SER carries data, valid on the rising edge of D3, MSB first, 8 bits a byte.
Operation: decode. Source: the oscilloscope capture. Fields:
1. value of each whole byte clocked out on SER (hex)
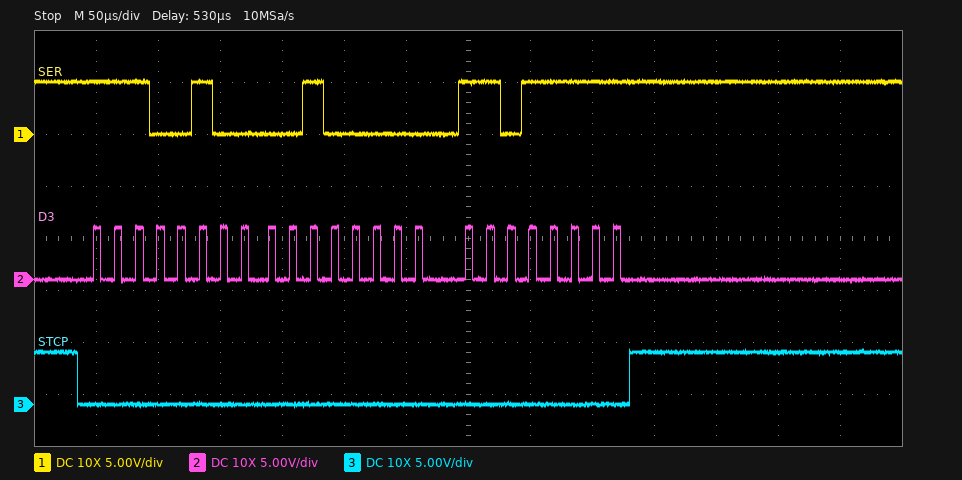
E4 20 DF
